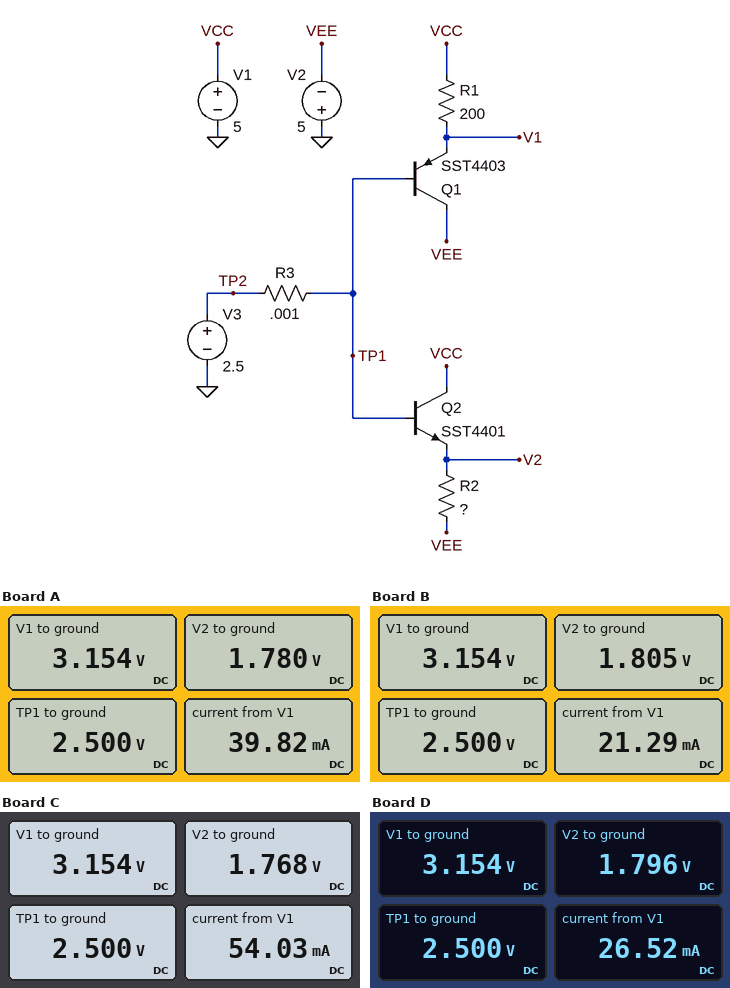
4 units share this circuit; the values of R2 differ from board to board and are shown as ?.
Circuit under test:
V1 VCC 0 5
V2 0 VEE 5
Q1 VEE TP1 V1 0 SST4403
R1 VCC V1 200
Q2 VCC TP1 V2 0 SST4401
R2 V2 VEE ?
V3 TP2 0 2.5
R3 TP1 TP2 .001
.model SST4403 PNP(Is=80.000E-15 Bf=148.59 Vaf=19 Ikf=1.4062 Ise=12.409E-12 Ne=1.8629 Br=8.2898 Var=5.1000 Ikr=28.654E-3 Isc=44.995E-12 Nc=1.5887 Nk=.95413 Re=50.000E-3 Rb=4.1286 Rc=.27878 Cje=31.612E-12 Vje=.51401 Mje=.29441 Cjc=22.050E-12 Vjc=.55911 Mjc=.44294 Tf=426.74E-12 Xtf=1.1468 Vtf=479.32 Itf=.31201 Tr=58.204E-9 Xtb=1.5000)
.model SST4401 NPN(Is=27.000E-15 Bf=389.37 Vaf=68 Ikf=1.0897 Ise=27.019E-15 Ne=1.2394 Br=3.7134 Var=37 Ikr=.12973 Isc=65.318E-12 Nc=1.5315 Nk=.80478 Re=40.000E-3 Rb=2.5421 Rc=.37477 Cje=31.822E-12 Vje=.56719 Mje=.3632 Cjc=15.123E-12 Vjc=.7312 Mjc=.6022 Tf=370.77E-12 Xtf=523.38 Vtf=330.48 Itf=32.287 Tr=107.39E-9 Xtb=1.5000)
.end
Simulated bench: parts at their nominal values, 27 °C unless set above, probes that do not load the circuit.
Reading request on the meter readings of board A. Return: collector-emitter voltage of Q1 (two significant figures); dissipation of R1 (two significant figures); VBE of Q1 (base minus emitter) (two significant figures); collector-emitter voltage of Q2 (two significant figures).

-8.2 V
17 mW
-650 mV
3.2 V
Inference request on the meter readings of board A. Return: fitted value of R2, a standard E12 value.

220 Ω
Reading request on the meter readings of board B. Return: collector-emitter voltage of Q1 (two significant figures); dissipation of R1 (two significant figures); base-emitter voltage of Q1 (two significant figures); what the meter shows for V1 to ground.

-8.2 V
17 mW
-650 mV
3.154 V
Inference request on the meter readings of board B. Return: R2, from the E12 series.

560 Ω
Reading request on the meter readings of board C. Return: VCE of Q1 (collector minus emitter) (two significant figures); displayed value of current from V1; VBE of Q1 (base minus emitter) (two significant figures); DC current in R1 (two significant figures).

-8.2 V
54.03 mA
-650 mV
9.2 mA
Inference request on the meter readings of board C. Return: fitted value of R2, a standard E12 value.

150 Ω
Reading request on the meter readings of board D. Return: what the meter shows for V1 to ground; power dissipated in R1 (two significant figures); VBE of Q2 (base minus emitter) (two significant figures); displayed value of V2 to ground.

3.154 V
17 mW
700 mV
1.796 V
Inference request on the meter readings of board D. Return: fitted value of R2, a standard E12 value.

390 Ω
